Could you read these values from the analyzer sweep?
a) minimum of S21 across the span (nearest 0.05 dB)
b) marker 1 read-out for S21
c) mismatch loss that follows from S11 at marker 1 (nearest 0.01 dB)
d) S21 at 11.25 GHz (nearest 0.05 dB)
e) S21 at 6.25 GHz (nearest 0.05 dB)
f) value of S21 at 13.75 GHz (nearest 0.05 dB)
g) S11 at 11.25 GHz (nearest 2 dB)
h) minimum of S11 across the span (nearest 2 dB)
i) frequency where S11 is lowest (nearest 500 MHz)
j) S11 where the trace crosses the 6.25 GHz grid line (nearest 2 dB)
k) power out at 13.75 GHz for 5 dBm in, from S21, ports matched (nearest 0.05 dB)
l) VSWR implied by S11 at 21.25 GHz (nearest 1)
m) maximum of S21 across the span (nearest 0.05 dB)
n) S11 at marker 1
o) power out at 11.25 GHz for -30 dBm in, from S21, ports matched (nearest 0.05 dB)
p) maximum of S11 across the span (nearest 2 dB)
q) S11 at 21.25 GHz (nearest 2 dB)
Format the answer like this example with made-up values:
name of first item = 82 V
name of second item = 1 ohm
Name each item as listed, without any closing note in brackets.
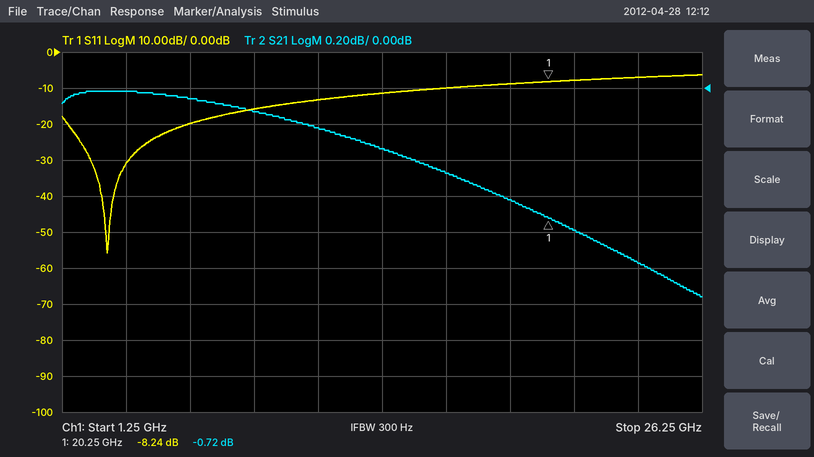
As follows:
minimum of S21 across the span = -1.15 dB
marker 1 read-out for S21 = -0.72 dB
mismatch loss that follows from S11 at marker 1 = 0.71 dB
S21 at 11.25 GHz = -0.20 dB
S21 at 6.25 GHz = -0.05 dB
value of S21 at 13.75 GHz = -0.35 dB
S11 at 11.25 GHz = -14 dB
minimum of S11 across the span = -56 dB
frequency where S11 is lowest = 3.0 GHz
S11 where the trace crosses the 6.25 GHz grid line = -20 dB
power out at 13.75 GHz for 5 dBm in, from S21, ports matched = 4.65 dBm
VSWR implied by S11 at 21.25 GHz = 2
maximum of S21 across the span = 0.00 dB
S11 at marker 1 = -8.24 dB
power out at 11.25 GHz for -30 dBm in, from S21, ports matched = -30.20 dBm
maximum of S11 across the span = -6 dB
S11 at 21.25 GHz = -8 dB
